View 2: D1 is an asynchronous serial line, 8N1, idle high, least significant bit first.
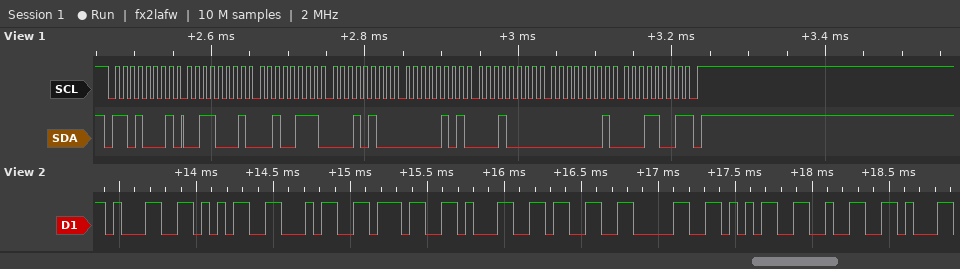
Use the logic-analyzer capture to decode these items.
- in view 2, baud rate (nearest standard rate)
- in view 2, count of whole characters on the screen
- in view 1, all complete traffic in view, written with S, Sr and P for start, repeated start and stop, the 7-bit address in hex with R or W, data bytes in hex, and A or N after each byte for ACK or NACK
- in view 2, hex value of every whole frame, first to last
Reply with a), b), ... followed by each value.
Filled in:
a) 19200 baud
b) 9
c) S 68R A 31 A 27 A 14 A 05 A 10 A 01 A 19 N P
d) 31 35 34 37 31 33 30 35 32
